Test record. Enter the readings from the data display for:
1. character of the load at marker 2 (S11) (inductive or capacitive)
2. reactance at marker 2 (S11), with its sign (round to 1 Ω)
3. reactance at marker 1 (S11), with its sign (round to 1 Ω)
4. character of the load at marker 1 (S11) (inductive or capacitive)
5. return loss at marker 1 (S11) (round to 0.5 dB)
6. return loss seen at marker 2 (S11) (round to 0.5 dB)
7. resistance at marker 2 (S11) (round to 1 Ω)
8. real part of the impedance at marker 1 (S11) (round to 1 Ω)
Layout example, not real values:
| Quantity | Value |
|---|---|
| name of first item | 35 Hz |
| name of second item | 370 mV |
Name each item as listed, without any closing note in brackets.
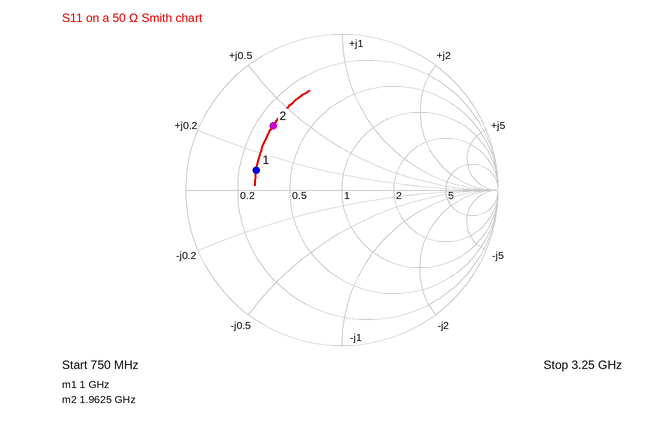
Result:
| Quantity | Value |
|---|---|
| character of the load at marker 2 (S11) | inductive |
| reactance at marker 2 (S11), with its sign | +18 Ω |
| reactance at marker 1 (S11), with its sign | +5 Ω |
| character of the load at marker 1 (S11) | inductive |
| return loss at marker 1 (S11) | 5.0 dB |
| return loss seen at marker 2 (S11) | 4.5 dB |
| resistance at marker 2 (S11) | 14 Ω |
| real part of the impedance at marker 1 (S11) | 14 Ω |
